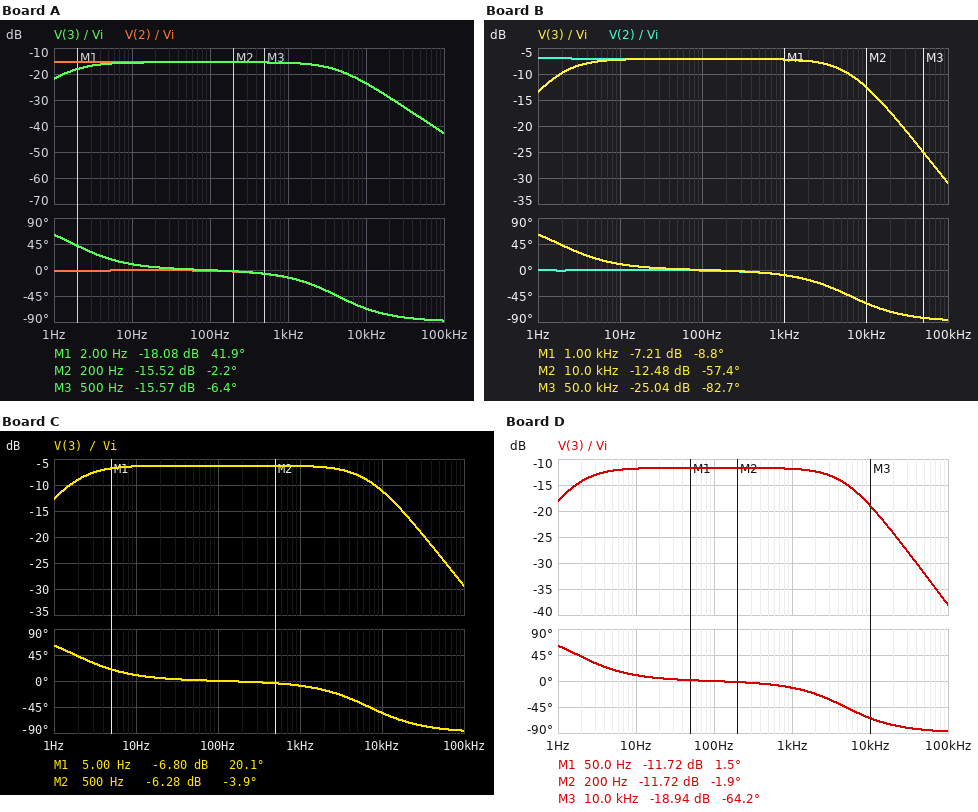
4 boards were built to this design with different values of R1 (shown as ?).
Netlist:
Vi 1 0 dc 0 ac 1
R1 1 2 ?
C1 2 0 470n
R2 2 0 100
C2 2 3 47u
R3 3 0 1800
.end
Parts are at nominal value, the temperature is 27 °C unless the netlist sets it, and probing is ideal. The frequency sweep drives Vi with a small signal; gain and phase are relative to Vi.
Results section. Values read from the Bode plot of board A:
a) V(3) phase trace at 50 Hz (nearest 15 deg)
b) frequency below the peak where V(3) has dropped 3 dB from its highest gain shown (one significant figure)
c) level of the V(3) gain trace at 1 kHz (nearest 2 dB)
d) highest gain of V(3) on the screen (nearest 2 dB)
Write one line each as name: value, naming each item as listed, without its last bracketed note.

V(3) phase trace at 50 Hz: 0 deg
frequency below the peak where V(3) has dropped 3 dB from its highest gain shown: 2 Hz
level of the V(3) gain trace at 1 kHz: -16 dB
highest gain of V(3) on the screen: -16 dB
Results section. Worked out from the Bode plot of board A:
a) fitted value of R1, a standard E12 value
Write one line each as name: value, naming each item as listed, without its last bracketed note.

fitted value of R1, a standard E12 value: 470 Ω
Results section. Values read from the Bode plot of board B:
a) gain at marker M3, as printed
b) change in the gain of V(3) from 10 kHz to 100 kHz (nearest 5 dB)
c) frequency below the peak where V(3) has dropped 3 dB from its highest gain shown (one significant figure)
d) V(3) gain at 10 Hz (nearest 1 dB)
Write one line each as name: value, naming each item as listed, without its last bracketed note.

gain at marker M3, as printed: -25.04 dB
change in the gain of V(3) from 10 kHz to 100 kHz: -20 dB
frequency below the peak where V(3) has dropped 3 dB from its highest gain shown: 2 Hz
V(3) gain at 10 Hz: -7 dB
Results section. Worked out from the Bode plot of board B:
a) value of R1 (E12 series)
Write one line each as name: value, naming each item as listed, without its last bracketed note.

value of R1: 120 Ω
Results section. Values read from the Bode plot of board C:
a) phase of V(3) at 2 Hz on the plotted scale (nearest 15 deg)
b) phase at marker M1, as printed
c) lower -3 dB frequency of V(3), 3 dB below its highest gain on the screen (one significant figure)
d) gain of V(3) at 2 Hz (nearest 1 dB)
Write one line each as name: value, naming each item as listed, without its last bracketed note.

phase of V(3) at 2 Hz on the plotted scale: 45 deg
phase at marker M1, as printed: 20.1 deg
lower -3 dB frequency of V(3), 3 dB below its highest gain on the screen: 2 Hz
gain of V(3) at 2 Hz: -9 dB
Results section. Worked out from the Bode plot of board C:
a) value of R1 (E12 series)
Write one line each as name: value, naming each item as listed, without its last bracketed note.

value of R1: 100 Ω
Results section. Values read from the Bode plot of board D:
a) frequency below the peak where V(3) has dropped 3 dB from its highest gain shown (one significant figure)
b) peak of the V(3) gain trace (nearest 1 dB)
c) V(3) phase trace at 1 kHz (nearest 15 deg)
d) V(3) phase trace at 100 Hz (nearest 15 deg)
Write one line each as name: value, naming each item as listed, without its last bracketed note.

frequency below the peak where V(3) has dropped 3 dB from its highest gain shown: 2 Hz
peak of the V(3) gain trace: -12 dB
V(3) phase trace at 1 kHz: -15 deg
V(3) phase trace at 100 Hz: 0 deg
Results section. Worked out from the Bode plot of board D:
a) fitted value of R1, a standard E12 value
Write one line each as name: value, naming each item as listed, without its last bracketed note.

fitted value of R1, a standard E12 value: 270 Ω
